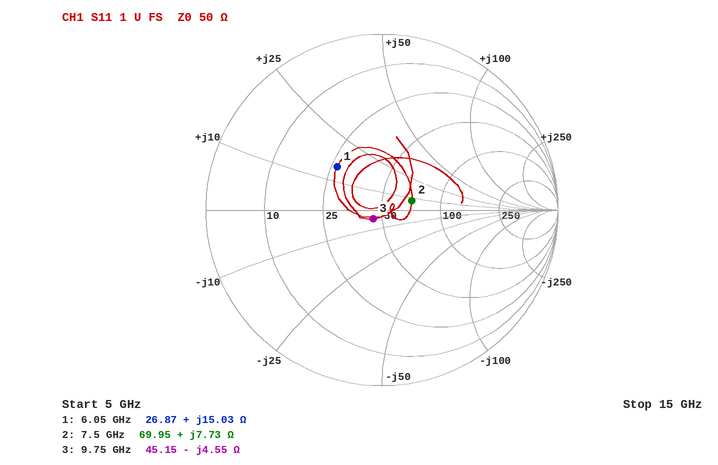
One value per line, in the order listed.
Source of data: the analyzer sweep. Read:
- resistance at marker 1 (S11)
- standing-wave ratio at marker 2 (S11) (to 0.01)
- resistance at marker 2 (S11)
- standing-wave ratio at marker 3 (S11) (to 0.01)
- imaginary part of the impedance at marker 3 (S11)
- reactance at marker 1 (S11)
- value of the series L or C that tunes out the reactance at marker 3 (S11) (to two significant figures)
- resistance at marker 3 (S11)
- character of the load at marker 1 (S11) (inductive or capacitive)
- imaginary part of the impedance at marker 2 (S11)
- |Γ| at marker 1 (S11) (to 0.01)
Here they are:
26.87 Ω
1.43
69.95 Ω
1.15
-4.55 Ω
+15.03 Ω
74 pH
45.15 Ω
inductive
+7.73 Ω
0.35
